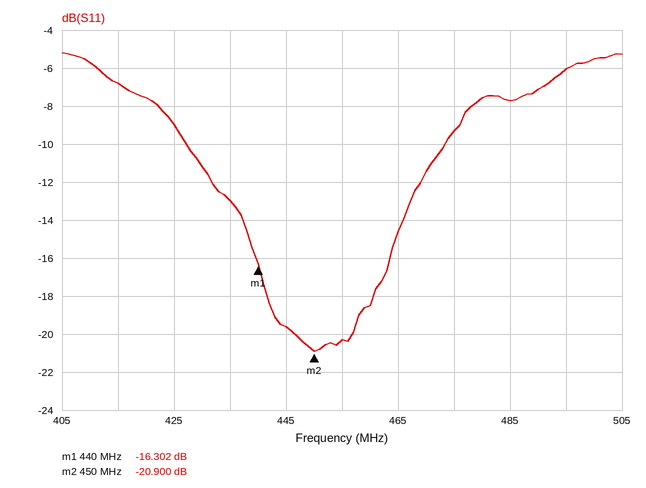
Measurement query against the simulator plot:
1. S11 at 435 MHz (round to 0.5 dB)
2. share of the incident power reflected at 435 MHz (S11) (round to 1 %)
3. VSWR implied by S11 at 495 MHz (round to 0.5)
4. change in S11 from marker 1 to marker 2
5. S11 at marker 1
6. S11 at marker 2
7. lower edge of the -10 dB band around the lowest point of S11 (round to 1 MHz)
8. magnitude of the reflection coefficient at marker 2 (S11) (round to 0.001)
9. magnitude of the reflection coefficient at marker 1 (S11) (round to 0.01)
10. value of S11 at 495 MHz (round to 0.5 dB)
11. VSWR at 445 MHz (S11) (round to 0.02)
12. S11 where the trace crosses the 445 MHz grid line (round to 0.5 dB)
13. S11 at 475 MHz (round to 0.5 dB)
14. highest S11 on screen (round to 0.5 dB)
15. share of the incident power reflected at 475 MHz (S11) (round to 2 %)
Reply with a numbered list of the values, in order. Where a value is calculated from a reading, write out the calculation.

1. -13.0 dB
2. 10^(-13/10) ≈ 5 %
3. |Γ| = 10^(-6/20) = 0.5012; VSWR = (1 + 0.5012)/(1 − 0.5012) ≈ 3.0
4. -20.9 − (-16.302) = -4.598 dB
5. -16.302 dB
6. -20.900 dB
7. 427 MHz
8. 10^(-20.9/20) ≈ 0.090
9. 10^(-16.302/20) ≈ 0.15
10. -6.0 dB
11. |Γ| = 10^(-19.5/20) = 0.1059; VSWR = (1 + 0.1059)/(1 − 0.1059) ≈ 1.24
12. -19.5 dB
13. -9.5 dB
14. -5.0 dB
15. 10^(-9.5/10) ≈ 11.2 %, so 12 % to the nearest 2 %
